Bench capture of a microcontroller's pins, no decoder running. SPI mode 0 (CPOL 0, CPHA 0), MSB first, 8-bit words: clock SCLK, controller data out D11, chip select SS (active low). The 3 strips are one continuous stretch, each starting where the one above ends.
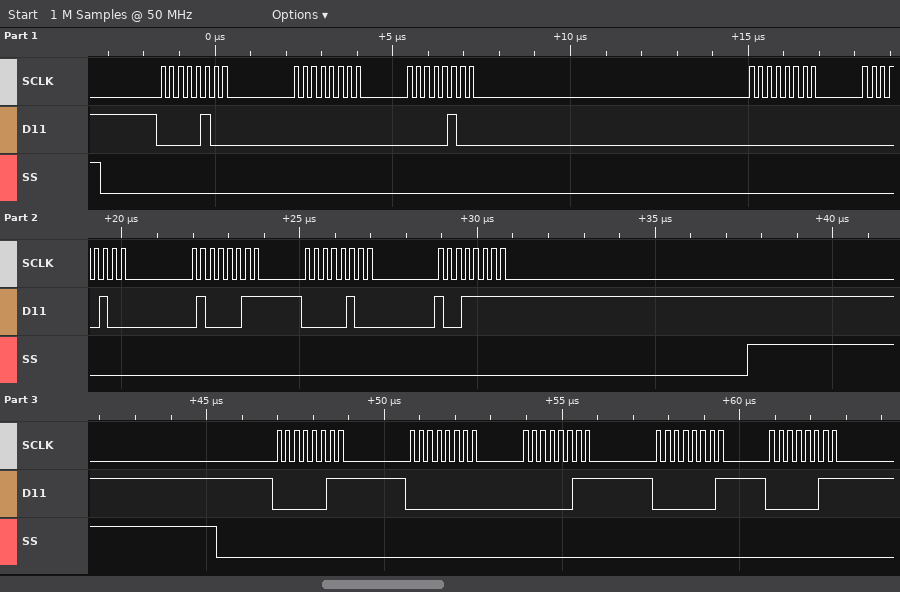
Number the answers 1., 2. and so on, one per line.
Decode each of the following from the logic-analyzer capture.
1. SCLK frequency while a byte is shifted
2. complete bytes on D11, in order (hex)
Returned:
1. 4 MHz
2. 04 00 04 00 04 43 04 9F 03 00 03 01 03
